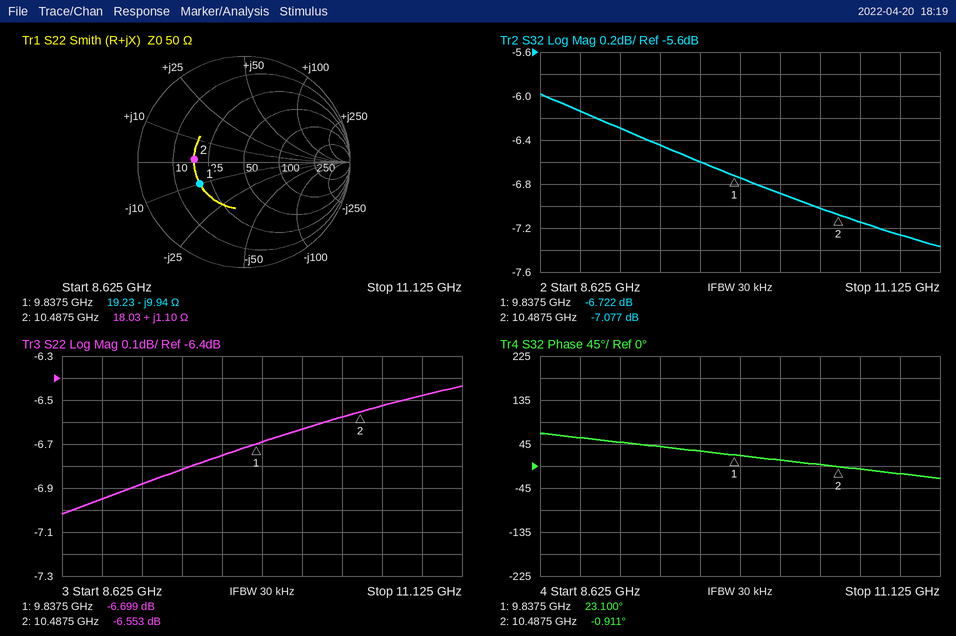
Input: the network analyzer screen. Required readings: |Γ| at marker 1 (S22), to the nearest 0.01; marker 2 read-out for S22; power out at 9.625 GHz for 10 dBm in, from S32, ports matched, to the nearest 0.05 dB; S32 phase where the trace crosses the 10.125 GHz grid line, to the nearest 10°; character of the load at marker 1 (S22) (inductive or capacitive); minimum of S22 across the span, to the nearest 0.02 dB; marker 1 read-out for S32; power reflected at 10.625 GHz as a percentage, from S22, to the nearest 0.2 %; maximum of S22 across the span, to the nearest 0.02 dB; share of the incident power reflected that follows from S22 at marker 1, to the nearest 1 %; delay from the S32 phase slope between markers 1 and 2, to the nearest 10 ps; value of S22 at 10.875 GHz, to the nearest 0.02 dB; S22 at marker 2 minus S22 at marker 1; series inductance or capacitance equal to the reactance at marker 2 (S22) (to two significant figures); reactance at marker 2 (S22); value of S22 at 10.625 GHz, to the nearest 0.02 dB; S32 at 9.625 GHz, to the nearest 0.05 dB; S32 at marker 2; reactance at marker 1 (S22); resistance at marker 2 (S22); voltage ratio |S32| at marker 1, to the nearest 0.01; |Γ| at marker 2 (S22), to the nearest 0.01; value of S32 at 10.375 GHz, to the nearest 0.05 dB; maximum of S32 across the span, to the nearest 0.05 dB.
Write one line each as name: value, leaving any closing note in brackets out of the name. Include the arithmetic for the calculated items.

|Γ| at marker 1 (S22), to the nearest 0.01: 0.46
marker 2 read-out for S22: -6.553 dB
power out at 9.625 GHz for 10 dBm in, from S32, ports matched, to the nearest 0.05 dB: 10 dBm + (-6.60 dB) = 3.40 dBm
S32 phase where the trace crosses the 10.125 GHz grid line, to the nearest 10°: 10°
character of the load at marker 1 (S22): capacitive
minimum of S22 across the span, to the nearest 0.02 dB: -7.02 dB
marker 1 read-out for S32: -6.722 dB
power reflected at 10.625 GHz as a percentage, from S22, to the nearest 0.2 %: 10^(-6.52/10) ≈ 22.3 %, so 22.2 % to the nearest 0.2 %
maximum of S22 across the span, to the nearest 0.02 dB: -6.44 dB
share of the incident power reflected that follows from S22 at marker 1, to the nearest 1 %: 10^(-6.699/10) ≈ 21 %
delay from the S32 phase slope between markers 1 and 2, to the nearest 10 ps: −(-0.911° − (23.1°))/(360° × 650 MHz) ≈ 103 ps, so 100 ps to the nearest 10 ps
value of S22 at 10.875 GHz, to the nearest 0.02 dB: -6.48 dB
S22 at marker 2 minus S22 at marker 1: -6.553 − (-6.699) = 0.146 dB
series inductance or capacitance equal to the reactance at marker 2 (S22): L = 1.1 Ω/(2π × 10.4875 GHz) ≈ 17 pH
reactance at marker 2: +1.10 Ω
value of S22 at 10.625 GHz, to the nearest 0.02 dB: -6.52 dB
S32 at 9.625 GHz, to the nearest 0.05 dB: -6.60 dB
S32 at marker 2: -7.077 dB
reactance at marker 1: -9.94 Ω
resistance at marker 2: 18.03 Ω
voltage ratio |S32| at marker 1, to the nearest 0.01: 10^(-6.722/20) ≈ 0.46
|Γ| at marker 2 (S22), to the nearest 0.01: 0.47
value of S32 at 10.375 GHz, to the nearest 0.05 dB: -7.00 dB
maximum of S32 across the span, to the nearest 0.05 dB: -6.00 dB
